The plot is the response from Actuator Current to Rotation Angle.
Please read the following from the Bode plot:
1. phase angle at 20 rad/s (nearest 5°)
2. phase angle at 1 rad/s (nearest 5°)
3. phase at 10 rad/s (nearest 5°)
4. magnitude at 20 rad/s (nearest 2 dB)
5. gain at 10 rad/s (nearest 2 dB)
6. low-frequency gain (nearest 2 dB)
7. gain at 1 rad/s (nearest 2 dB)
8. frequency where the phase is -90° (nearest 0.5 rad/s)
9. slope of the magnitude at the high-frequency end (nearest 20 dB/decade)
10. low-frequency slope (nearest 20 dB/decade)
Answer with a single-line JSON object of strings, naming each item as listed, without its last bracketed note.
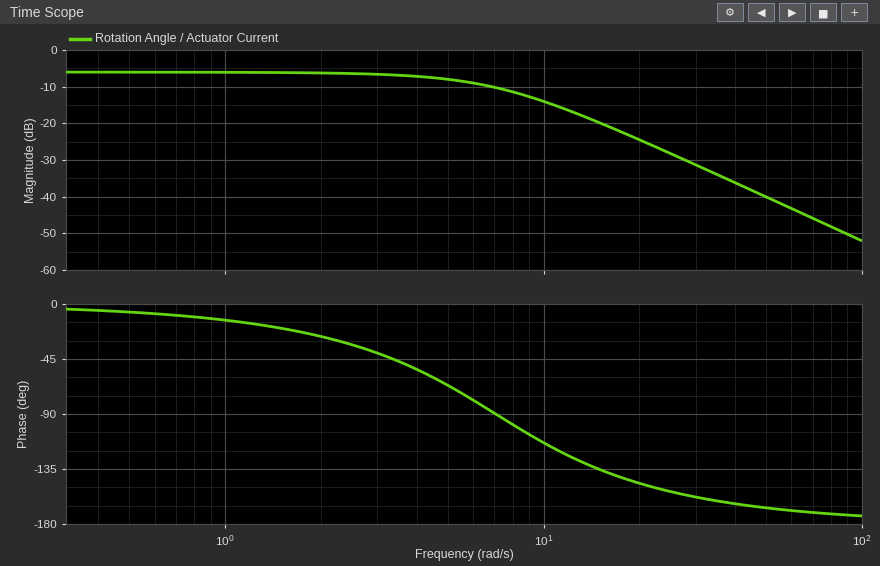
{"phase angle at 20 rad/s": "-145°", "phase angle at 1 rad/s": "-15°", "phase at 10 rad/s": "-115°", "magnitude at 20 rad/s": "-24 dB", "gain at 10 rad/s": "-14 dB", "low-frequency gain": "-6 dB", "gain at 1 rad/s": "-6 dB", "frequency where the phase is -90°": "7.0 rad/s", "slope of the magnitude at the high-frequency end": "-40 dB/decade", "low-frequency slope": "0 dB/decade"}
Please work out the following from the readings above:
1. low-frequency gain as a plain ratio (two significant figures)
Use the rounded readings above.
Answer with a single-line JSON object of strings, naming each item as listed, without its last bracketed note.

{"low-frequency gain as a plain ratio": "0.50"}
